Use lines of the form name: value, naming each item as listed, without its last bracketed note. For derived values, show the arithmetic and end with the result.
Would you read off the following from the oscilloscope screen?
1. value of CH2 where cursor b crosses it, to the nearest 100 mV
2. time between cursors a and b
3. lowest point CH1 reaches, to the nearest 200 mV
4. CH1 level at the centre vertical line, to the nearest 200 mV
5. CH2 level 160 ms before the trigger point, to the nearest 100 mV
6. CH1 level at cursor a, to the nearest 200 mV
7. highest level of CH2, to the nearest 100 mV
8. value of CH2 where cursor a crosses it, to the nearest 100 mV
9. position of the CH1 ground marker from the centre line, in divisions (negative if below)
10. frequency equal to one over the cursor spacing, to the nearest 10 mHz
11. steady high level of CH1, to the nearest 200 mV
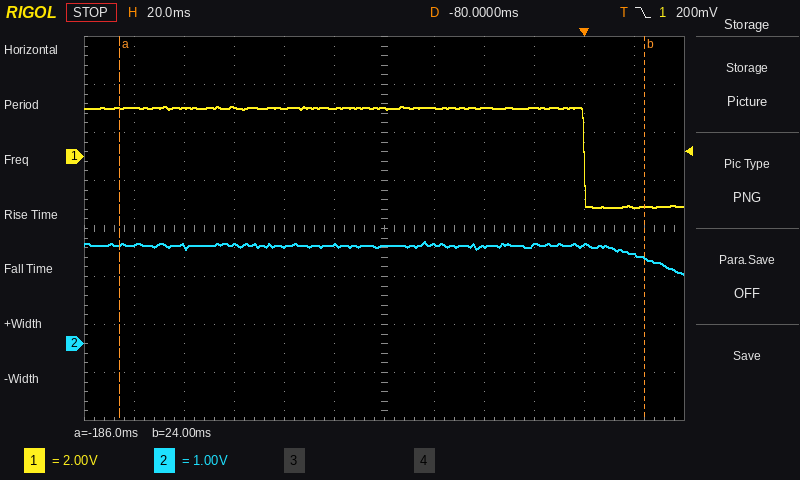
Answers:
value of CH2 where cursor b crosses it, to the nearest 100 mV: 1.8 V
time between cursors a and b: 24 ms − (-186 ms) = 210 ms
lowest point CH1 reaches, to the nearest 200 mV: -2.2 V
CH1 level at the centre vertical line, to the nearest 200 mV: 2.0 V
CH2 level 160 ms before the trigger point, to the nearest 100 mV: 2.0 V
CH1 level at cursor a, to the nearest 200 mV: 2.0 V
highest level of CH2, to the nearest 100 mV: 2.1 V
value of CH2 where cursor a crosses it, to the nearest 100 mV: 2.1 V
position of the CH1 ground marker from the centre line, in divisions: +1.5 div
frequency equal to one over the cursor spacing, to the nearest 10 mHz: 1 / 210 ms ≈ 4.76 Hz
steady high level of CH1, to the nearest 200 mV: 2.0 V
